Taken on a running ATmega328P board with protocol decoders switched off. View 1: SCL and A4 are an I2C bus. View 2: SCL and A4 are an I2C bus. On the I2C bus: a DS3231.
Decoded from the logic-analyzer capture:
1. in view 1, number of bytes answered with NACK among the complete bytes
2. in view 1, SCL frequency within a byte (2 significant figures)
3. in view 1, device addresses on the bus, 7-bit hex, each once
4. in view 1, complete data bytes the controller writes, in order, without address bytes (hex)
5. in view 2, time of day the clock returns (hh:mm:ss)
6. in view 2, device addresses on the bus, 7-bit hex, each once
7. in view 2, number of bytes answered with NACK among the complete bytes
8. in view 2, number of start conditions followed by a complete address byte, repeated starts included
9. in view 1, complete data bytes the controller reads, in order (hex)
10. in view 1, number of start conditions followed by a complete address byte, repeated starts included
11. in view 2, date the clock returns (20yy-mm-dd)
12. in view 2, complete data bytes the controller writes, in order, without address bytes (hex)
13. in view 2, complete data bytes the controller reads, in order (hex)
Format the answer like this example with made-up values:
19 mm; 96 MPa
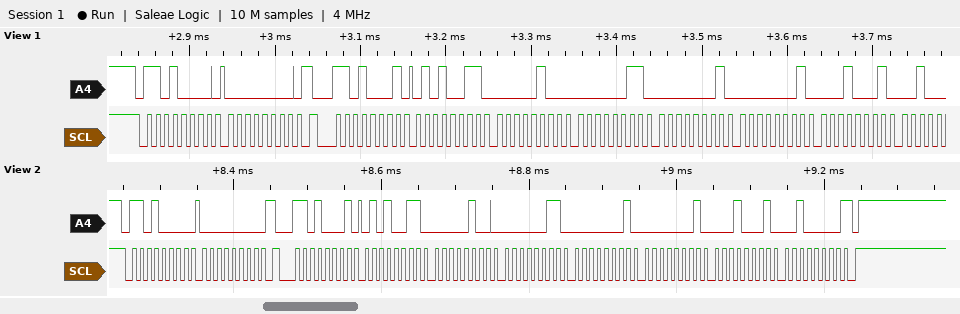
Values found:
0; 100 kHz; 0x68; 00; 03:04:53; 0x68; 1; 2; 53 04 03 01 01 11; 2; 2020-11-01; 00; 53 04 03 01 01 11 20
